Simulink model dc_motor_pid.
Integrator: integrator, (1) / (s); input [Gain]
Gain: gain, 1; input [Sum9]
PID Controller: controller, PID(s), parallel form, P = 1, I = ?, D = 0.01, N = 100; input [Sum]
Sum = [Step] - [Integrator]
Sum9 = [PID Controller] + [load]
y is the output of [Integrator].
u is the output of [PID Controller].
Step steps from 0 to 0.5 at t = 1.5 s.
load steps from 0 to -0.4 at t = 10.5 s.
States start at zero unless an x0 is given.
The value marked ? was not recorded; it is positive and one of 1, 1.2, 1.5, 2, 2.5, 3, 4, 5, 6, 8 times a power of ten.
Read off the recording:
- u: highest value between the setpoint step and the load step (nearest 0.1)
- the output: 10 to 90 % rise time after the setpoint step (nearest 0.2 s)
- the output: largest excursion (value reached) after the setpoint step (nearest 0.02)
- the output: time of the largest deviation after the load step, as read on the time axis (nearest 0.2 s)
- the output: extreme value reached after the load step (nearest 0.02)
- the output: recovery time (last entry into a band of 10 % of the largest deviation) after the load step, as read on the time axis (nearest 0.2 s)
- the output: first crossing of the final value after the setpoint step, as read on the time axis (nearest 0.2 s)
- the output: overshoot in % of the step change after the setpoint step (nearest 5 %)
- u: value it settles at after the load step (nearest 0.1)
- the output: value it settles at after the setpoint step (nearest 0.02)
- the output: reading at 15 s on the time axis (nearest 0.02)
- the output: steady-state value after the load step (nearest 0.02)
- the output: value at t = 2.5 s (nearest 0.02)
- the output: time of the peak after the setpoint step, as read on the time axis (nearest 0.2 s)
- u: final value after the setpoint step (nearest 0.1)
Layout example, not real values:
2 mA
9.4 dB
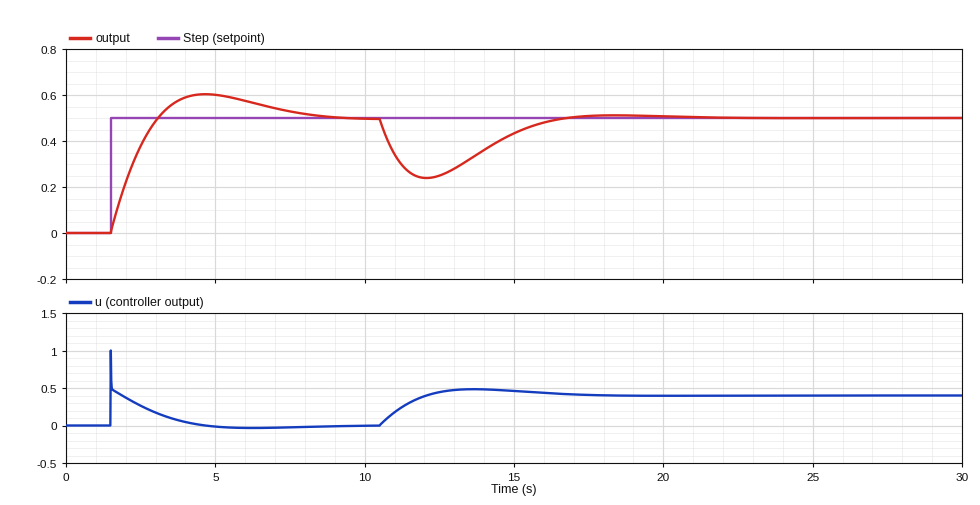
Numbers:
1.0
1.2 s
0.60
12.0 s
0.24
15.8 s
3.0 s
20 %
0.4
0.50
0.44
0.50
0.38
4.6 s
0.0
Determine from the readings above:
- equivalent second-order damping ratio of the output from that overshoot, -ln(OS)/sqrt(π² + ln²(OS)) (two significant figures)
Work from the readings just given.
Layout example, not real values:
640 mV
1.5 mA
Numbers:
0.46
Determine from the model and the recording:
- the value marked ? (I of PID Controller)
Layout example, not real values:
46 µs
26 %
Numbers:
0.5
